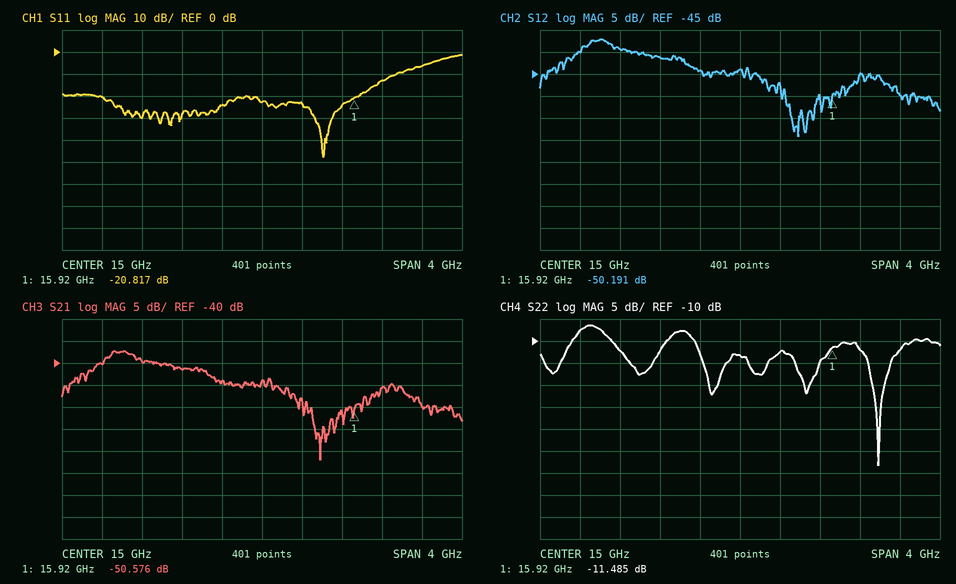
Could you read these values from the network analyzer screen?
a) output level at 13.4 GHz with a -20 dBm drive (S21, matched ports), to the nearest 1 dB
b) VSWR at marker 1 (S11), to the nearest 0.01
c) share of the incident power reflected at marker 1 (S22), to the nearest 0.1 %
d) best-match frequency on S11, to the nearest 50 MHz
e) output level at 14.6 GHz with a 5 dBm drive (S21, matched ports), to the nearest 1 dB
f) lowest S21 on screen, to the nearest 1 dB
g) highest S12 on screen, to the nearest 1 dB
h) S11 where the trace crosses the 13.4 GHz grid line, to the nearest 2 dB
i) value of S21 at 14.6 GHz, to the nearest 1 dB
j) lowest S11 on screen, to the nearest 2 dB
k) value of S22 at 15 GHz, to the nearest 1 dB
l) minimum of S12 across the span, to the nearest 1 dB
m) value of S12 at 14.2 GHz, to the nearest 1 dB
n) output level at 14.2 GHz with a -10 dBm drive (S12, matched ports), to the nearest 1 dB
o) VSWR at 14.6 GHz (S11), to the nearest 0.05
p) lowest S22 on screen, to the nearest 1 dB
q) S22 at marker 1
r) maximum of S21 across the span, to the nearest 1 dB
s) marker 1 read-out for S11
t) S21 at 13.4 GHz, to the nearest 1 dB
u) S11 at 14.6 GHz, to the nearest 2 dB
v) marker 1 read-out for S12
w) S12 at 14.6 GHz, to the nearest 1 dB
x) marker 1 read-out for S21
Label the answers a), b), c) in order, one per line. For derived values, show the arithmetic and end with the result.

a) -20 dBm + (-40 dB) = -60 dBm
b) (1 + 0.0910)/(1 − 0.0910) ≈ 1.20
c) 10^(-11.485/10) ≈ 7.1 %
d) 15.60 GHz
e) 5 dBm + (-44 dB) = -39 dBm
f) -62 dB
g) -37 dB
h) -20 dB
i) -44 dB
j) -48 dB
k) -13 dB
l) -59 dB
m) -41 dB
n) -10 dBm + (-41 dB) = -51 dBm
o) |Γ| = 10^(-24/20) = 0.0631; VSWR = (1 + 0.0631)/(1 − 0.0631) ≈ 1.13, so 1.15 to the nearest 0.05
p) -38 dB
q) -11.485 dB
r) -37 dB
s) -20.817 dB
t) -40 dB
u) -24 dB
v) -50.191 dB
w) -44 dB
x) -50.576 dB
